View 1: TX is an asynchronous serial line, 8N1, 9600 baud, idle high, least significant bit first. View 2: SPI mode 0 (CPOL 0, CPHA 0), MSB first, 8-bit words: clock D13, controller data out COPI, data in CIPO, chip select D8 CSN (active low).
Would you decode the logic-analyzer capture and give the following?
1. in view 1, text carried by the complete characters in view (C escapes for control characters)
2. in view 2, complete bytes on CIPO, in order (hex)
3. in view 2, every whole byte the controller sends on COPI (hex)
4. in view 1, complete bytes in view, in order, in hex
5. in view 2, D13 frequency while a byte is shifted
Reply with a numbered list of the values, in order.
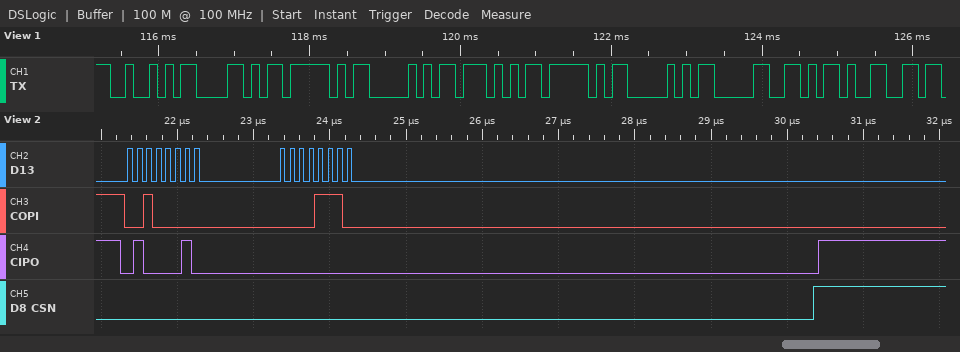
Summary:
1. "RX_PW_P0-"
2. 0x42 0x00
3. 0x20 0x0E
4. 52 58 5F 50 57 5F 50 30 2D
5. 8 MHz
